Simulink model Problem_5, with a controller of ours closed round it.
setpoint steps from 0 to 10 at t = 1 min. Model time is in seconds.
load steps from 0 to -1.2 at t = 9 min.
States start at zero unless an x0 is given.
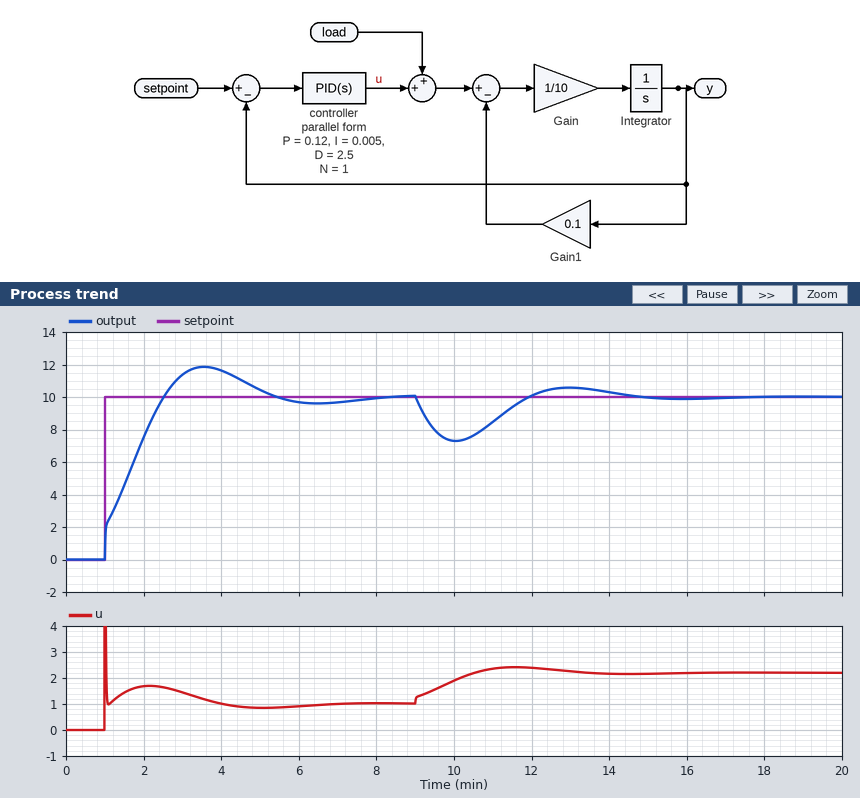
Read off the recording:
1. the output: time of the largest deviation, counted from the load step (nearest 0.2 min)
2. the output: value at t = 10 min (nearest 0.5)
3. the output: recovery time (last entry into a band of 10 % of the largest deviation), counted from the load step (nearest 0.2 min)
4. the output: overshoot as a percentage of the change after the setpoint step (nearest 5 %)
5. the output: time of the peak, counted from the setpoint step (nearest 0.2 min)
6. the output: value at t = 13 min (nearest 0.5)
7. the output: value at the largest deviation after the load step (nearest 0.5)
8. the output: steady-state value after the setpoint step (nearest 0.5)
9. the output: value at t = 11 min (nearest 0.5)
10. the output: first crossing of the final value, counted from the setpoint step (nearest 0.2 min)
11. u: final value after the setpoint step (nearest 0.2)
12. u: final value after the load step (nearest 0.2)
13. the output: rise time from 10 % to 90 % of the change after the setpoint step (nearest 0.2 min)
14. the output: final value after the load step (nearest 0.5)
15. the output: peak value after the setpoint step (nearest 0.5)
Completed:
1.0 min
7.5
5.0 min
20 %
2.6 min
10.5
7.5
10.0
8.5
1.6 min
1.0
2.2
1.2 min
10.0
12.0
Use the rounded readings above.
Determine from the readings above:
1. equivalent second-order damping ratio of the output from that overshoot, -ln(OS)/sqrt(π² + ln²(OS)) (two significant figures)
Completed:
0.46
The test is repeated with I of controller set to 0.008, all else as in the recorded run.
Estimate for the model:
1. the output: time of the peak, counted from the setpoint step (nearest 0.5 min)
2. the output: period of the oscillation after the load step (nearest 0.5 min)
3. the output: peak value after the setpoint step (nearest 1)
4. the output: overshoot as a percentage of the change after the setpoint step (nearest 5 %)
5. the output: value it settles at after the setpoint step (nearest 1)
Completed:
2.0 min
4.5 min
13
25 %
10
